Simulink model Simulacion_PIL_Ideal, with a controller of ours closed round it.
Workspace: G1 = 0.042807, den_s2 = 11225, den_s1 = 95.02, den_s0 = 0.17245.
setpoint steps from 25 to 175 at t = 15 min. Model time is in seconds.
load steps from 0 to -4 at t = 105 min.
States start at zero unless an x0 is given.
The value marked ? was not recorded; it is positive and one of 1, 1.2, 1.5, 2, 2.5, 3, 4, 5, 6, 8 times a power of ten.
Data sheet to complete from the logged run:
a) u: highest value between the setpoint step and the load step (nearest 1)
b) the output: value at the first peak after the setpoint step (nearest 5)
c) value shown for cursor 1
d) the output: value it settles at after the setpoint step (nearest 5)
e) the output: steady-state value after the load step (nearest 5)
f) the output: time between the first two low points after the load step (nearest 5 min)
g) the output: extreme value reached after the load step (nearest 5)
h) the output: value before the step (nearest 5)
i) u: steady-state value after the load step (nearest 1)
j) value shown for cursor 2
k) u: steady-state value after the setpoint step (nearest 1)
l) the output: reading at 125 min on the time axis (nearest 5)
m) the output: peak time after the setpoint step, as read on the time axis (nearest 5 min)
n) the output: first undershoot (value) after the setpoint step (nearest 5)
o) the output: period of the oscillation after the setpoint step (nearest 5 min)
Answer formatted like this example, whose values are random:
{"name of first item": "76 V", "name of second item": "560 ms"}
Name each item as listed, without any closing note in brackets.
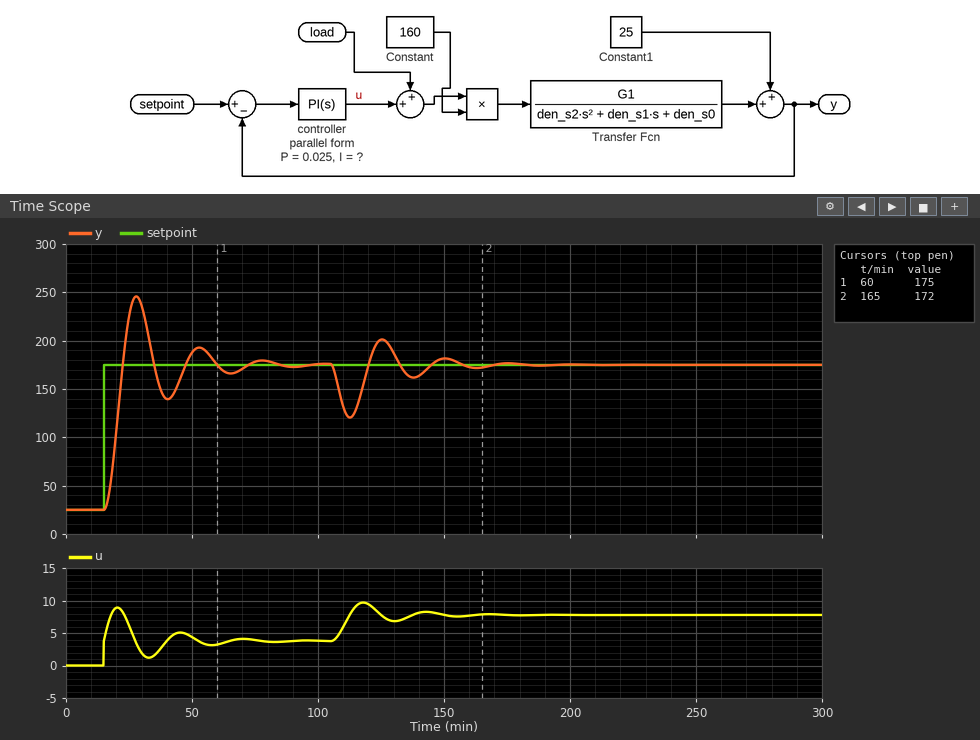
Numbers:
{"u: highest value between the setpoint step and the load step": "9", "the output: value at the first peak after the setpoint step": "245", "value shown for cursor 1": "175", "the output: value it settles at after the setpoint step": "175", "the output: steady-state value after the load step": "175", "the output: time between the first two low points after the load step": "25 min", "the output: extreme value reached after the load step": "120", "the output: value before the step": "25", "u: steady-state value after the load step": "8", "value shown for cursor 2": "172", "u: steady-state value after the setpoint step": "4", "the output: reading at 125 min on the time axis": "200", "the output: peak time after the setpoint step, as read on the time axis": "30 min", "the output: first undershoot (value) after the setpoint step": "140", "the output: period of the oscillation after the setpoint step": "25 min"}
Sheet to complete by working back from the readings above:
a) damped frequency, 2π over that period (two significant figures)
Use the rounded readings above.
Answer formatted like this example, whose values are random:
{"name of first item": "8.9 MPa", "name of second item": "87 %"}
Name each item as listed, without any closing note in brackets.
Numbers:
{"damped frequency, 2π over that period": "0.25 rad/min"}
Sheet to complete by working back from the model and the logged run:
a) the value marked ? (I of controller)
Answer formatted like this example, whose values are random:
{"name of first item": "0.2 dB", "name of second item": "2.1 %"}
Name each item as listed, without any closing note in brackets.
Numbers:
{"the value marked ?": "0.0002"}
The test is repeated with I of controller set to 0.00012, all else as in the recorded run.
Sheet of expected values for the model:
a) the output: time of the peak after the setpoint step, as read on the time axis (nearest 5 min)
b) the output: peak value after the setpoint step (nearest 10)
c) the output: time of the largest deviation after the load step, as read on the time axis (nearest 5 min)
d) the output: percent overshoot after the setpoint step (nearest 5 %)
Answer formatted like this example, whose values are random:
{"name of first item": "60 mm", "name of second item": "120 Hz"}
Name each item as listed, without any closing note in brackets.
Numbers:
{"the output: time of the peak after the setpoint step, as read on the time axis": "30 min", "the output: peak value after the setpoint step": "210", "the output: time of the largest deviation after the load step, as read on the time axis": "115 min", "the output: percent overshoot after the setpoint step": "25 %"}
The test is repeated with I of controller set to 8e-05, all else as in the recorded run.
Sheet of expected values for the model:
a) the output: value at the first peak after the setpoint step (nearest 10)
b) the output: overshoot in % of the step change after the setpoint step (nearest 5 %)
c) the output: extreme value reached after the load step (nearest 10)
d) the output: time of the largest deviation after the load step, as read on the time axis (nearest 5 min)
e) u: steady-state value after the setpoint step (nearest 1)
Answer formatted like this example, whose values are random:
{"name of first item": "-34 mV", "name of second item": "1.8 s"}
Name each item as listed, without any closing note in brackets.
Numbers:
{"the output: value at the first peak after the setpoint step": "190", "the output: overshoot in % of the step change after the setpoint step": "10 %", "the output: extreme value reached after the load step": "110", "the output: time of the largest deviation after the load step, as read on the time axis": "115 min", "u: steady-state value after the setpoint step": "4"}
